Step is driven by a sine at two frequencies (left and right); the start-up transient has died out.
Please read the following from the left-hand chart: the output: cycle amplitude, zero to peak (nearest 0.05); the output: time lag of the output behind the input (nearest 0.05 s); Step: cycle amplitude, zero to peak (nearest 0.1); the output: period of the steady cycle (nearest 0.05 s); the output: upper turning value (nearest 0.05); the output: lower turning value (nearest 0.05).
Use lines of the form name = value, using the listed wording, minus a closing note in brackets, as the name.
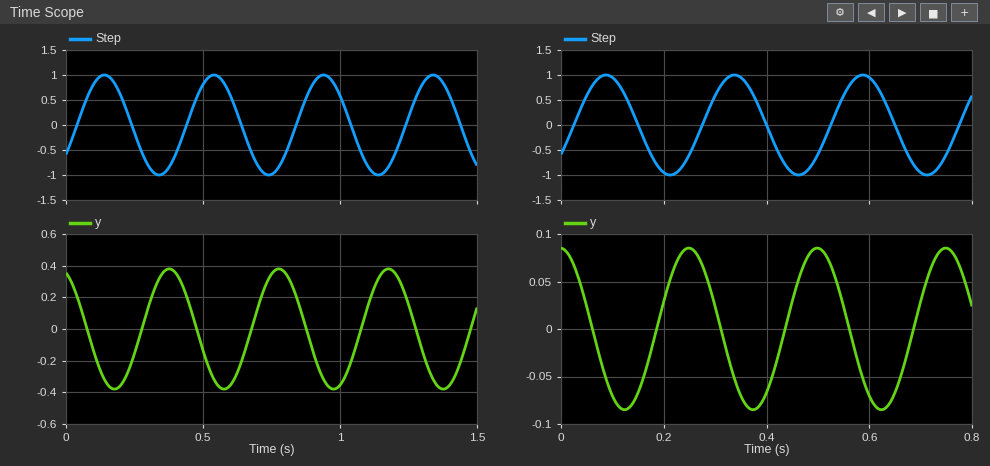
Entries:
the output: cycle amplitude, zero to peak = 0.40
the output: time lag of the output behind the input = 0.25 s
Step: cycle amplitude, zero to peak = 1.0
the output: period of the steady cycle = 0.40 s
the output: upper turning value = 0.40
the output: lower turning value = -0.40
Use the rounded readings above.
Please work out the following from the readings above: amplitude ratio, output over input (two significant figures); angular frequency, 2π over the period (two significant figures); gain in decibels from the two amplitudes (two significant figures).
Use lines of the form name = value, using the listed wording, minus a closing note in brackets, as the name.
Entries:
amplitude ratio, output over input = 0.40
angular frequency, 2π over the period = 16 rad/s
gain in decibels from the two amplitudes = -8.0 dB
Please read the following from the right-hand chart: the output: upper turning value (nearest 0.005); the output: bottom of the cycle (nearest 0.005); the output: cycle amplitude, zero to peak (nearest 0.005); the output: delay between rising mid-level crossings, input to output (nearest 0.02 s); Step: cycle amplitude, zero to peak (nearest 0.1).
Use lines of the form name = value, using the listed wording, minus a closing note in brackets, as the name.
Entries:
the output: upper turning value = 0.085
the output: bottom of the cycle = -0.085
the output: cycle amplitude, zero to peak = 0.085
the output: delay between rising mid-level crossings, input to output = 0.16 s
Step: cycle amplitude, zero to peak = 1.0
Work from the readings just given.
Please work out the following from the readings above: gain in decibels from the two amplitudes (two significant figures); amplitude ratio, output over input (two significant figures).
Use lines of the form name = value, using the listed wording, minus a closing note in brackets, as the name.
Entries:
gain in decibels from the two amplitudes = -21 dB
amplitude ratio, output over input = 0.085
